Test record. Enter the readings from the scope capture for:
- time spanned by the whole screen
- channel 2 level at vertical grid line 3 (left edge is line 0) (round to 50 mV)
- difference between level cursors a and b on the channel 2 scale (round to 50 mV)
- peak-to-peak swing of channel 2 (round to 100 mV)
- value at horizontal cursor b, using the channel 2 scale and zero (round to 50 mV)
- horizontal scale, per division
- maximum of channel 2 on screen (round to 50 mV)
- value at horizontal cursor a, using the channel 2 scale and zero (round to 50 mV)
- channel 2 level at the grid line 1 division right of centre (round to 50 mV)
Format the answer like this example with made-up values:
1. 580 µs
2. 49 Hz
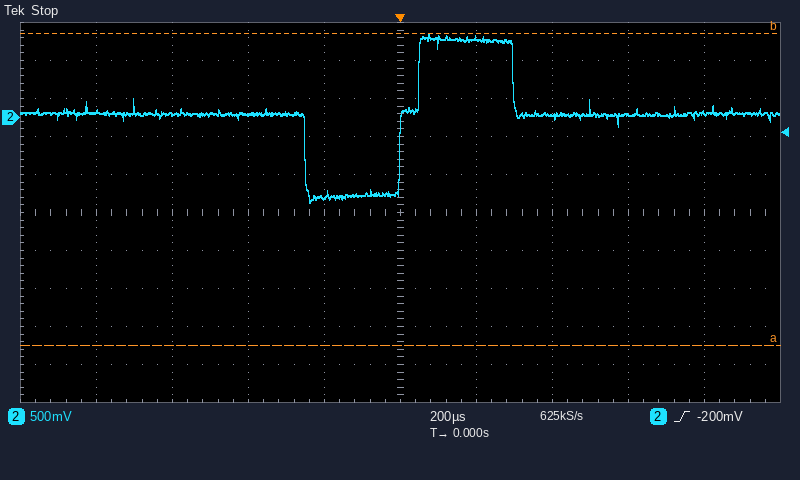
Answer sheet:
1. 2 ms
2. 50 mV
3. 4.10 V
4. 2.20 V
5. 1.10 V
6. 200 µs
7. 1.10 V
8. -3.00 V
9. 1.05 V
